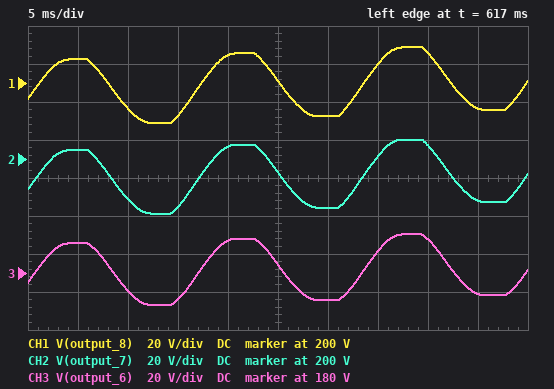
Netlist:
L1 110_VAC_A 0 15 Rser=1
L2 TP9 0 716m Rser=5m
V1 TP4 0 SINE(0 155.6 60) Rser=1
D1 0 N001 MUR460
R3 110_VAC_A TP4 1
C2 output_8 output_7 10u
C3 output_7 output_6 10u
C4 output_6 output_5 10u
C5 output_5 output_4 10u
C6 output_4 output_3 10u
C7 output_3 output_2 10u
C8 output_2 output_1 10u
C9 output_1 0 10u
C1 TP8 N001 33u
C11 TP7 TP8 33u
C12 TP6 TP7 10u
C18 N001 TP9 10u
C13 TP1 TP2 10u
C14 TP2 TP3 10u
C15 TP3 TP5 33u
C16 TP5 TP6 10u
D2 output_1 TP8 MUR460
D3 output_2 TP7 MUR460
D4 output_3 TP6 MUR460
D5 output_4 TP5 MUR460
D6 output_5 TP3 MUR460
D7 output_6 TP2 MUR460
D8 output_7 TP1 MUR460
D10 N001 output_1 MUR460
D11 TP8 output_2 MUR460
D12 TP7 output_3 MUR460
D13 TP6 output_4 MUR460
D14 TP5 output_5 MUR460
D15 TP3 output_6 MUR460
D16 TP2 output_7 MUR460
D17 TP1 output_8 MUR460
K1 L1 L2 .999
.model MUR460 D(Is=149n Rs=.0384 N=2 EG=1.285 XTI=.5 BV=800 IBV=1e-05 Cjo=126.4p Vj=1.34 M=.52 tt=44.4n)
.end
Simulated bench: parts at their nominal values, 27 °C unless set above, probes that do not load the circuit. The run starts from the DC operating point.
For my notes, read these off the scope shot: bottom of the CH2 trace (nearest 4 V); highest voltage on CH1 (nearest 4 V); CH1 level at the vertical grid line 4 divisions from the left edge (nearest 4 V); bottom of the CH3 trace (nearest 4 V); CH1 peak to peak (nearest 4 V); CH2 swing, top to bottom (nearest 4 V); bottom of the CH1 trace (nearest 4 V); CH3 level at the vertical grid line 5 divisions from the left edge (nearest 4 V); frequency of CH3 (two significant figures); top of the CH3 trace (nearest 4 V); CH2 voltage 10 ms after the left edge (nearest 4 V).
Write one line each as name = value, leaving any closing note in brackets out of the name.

bottom of the CH2 trace = 172 V
highest voltage on CH1 = 220 V
CH1 level at the vertical grid line 4 divisions from the left edge = 216 V
bottom of the CH3 trace = 164 V
CH1 peak to peak = 40 V
CH2 swing, top to bottom = 40 V
bottom of the CH1 trace = 180 V
CH3 level at the vertical grid line 5 divisions from the left edge = 184 V
frequency of CH3 = 61 Hz
top of the CH3 trace = 200 V
CH2 voltage 10 ms after the left edge = 180 V
